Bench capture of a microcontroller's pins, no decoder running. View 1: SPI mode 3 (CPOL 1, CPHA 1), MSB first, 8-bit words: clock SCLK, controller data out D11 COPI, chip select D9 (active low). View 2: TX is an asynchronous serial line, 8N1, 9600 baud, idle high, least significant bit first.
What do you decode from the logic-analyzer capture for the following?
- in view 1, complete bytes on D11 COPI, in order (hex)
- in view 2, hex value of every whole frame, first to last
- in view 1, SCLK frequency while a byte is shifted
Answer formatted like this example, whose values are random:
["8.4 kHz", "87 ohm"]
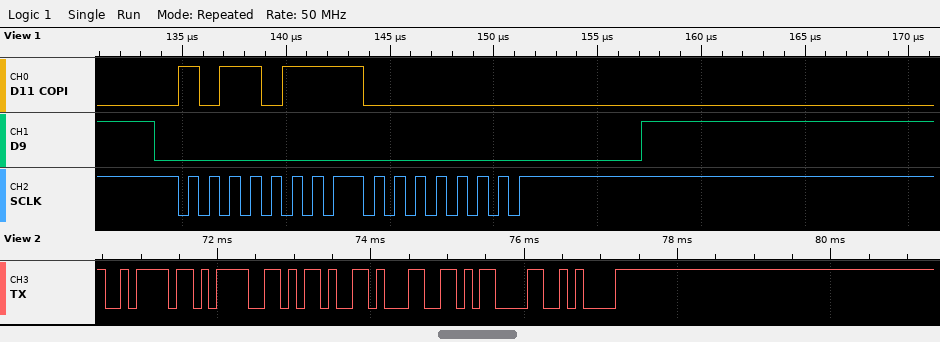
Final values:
["B7 00", "7A 3D 2D 31 0D 0A", "1 MHz"]
